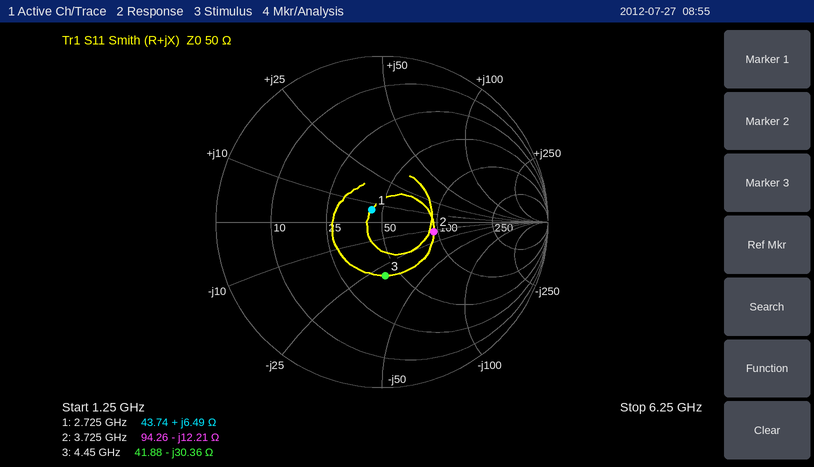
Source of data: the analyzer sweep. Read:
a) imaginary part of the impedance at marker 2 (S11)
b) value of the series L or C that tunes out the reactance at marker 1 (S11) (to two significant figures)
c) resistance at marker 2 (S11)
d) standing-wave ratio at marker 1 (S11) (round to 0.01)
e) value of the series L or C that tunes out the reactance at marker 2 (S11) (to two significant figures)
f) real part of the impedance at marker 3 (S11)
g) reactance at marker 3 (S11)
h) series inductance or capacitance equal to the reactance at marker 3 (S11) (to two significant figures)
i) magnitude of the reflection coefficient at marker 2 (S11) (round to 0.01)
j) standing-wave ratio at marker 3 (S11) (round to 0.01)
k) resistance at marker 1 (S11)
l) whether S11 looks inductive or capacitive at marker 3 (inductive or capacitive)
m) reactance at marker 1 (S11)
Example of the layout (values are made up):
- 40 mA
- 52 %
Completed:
- -12.21 Ω
- 9.0 pF
- 94.26 Ω
- 1.21
- 520 pH
- 41.88 Ω
- -30.36 Ω
- 1.2 pF
- 0.32
- 1.96
- 43.74 Ω
- capacitive
- +6.49 Ω
